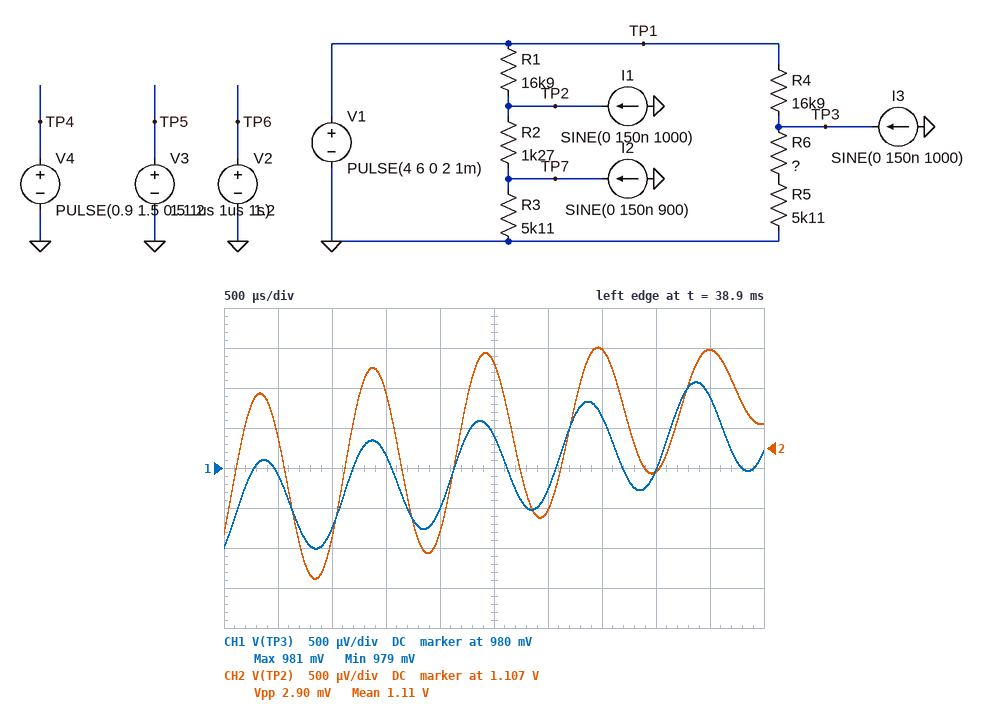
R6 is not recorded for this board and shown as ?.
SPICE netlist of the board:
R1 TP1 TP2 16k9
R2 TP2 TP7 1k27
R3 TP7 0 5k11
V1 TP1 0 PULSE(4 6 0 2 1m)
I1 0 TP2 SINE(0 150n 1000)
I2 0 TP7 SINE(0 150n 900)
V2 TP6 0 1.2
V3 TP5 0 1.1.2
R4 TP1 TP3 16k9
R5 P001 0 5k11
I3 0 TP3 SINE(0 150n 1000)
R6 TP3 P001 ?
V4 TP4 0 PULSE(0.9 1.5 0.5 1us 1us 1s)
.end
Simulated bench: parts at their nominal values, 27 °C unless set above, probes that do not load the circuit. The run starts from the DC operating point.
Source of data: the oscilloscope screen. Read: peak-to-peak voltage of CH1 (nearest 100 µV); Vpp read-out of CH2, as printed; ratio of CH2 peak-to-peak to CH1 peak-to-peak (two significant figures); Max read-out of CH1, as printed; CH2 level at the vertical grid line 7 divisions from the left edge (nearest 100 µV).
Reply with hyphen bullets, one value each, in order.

- 2.1 mV
- 2.90 mV
- 1.4
- 981 mV
- 1.1087 V
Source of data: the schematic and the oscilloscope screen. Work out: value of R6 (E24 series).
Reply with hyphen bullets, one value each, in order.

- 300 Ω
